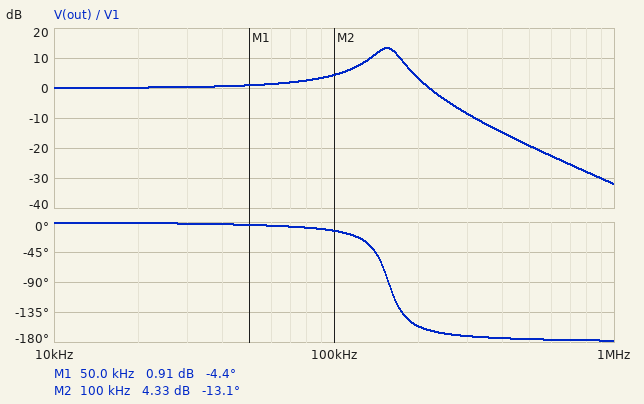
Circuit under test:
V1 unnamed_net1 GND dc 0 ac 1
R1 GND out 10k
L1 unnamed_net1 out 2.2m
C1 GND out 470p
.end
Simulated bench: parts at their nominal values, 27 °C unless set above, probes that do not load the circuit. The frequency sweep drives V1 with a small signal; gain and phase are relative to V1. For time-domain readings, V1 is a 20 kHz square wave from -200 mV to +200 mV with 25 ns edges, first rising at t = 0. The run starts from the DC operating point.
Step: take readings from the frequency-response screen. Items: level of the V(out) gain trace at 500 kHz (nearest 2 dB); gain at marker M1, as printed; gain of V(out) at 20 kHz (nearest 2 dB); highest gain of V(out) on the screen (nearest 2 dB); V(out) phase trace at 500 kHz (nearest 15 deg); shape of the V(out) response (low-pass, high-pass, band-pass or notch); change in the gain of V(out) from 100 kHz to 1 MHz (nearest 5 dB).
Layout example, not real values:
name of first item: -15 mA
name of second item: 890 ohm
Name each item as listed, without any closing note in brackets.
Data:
level of the V(out) gain trace at 500 kHz: -20 dB
gain at marker M1, as printed: 0.91 dB
gain of V(out) at 20 kHz: 0 dB
highest gain of V(out) on the screen: 14 dB
V(out) phase trace at 500 kHz: -180 deg
shape of the V(out) response: low-pass
change in the gain of V(out) from 100 kHz to 1 MHz: -35 dB
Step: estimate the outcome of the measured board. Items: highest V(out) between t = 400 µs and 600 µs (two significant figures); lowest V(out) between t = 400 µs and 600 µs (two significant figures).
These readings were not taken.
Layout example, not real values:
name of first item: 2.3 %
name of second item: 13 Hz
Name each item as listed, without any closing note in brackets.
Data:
highest V(out) between t = 400 µs and 600 µs: 470 mV
lowest V(out) between t = 400 µs and 600 µs: -470 mV
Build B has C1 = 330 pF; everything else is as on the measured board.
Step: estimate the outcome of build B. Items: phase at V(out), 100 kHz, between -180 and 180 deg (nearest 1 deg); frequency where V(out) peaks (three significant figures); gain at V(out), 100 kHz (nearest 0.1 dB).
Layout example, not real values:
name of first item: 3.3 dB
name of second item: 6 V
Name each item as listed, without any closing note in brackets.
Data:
phase at V(out), 100 kHz, between -180 and 180 deg: -11 deg
frequency where V(out) peaks: 184 kHz
gain at V(out), 100 kHz: 2.8 dB
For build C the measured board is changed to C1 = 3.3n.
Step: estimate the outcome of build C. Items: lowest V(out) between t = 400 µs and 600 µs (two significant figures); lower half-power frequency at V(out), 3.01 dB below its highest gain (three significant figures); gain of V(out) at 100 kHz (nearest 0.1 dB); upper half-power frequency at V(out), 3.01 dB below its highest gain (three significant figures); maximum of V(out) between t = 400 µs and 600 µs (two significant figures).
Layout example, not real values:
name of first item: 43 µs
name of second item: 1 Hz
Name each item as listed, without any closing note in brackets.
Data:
lowest V(out) between t = 400 µs and 600 µs: -1.2 V
lower half-power frequency at V(out), 3.01 dB below its highest gain: 56.5 kHz
gain of V(out) at 100 kHz: -5.4 dB
upper half-power frequency at V(out), 3.01 dB below its highest gain: 61.3 kHz
maximum of V(out) between t = 400 µs and 600 µs: 1.2 V
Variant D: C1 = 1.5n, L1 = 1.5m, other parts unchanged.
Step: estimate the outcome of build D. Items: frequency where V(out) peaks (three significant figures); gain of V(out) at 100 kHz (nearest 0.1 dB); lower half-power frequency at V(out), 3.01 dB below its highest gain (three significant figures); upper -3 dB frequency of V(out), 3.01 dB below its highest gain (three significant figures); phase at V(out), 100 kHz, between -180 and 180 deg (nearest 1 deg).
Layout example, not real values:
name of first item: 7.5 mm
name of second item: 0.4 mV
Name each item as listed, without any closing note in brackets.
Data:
frequency where V(out) peaks: 106 kHz
gain of V(out) at 100 kHz: 16.7 dB
lower half-power frequency at V(out), 3.01 dB below its highest gain: 100 kHz
upper -3 dB frequency of V(out), 3.01 dB below its highest gain: 111 kHz
phase at V(out), 100 kHz, between -180 and 180 deg: -40 deg
